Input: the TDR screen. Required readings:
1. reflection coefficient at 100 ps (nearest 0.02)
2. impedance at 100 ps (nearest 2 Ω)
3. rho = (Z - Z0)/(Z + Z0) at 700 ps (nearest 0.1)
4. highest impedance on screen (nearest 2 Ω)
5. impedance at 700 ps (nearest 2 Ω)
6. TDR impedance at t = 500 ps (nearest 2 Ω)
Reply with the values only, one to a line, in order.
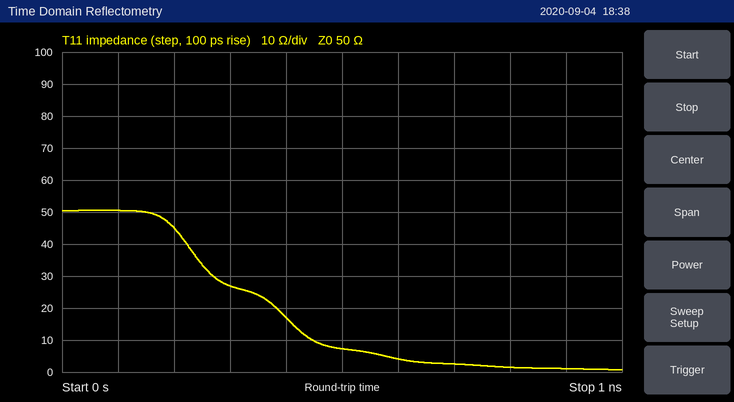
0.00
50 Ω
-0.9
50 Ω
2 Ω
8 Ω
